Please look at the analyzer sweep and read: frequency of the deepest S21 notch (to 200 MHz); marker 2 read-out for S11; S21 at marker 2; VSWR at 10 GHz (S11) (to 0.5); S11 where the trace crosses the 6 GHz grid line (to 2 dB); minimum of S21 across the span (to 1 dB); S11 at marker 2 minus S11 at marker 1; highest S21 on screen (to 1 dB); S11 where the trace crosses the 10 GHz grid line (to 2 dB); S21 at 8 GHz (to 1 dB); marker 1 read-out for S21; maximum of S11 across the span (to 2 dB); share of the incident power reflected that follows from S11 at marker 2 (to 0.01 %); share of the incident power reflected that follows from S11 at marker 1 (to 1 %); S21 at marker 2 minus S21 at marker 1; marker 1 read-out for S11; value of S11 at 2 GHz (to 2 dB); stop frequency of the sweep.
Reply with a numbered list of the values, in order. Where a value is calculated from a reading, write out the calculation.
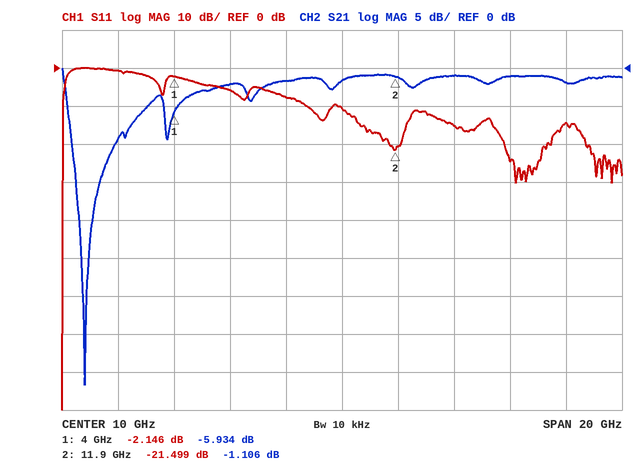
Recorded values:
1. 800 MHz
2. -21.499 dB
3. -1.106 dB
4. |Γ| = 10^(-10/20) = 0.3162; VSWR = (1 + 0.3162)/(1 − 0.3162) ≈ 1.92, so 2.0 to the nearest 0.5
5. -6 dB
6. -42 dB
7. -21.499 − (-2.146) = -19.353 dB
8. 0 dB
9. -10 dB
10. -2 dB
11. -5.934 dB
12. 0 dB
13. 10^(-21.499/10) ≈ 0.71 %
14. 10^(-2.146/10) ≈ 61 %
15. -1.106 − (-5.934) = 4.828 dB
16. -2.146 dB
17. 0 dB
18. 20 GHz
